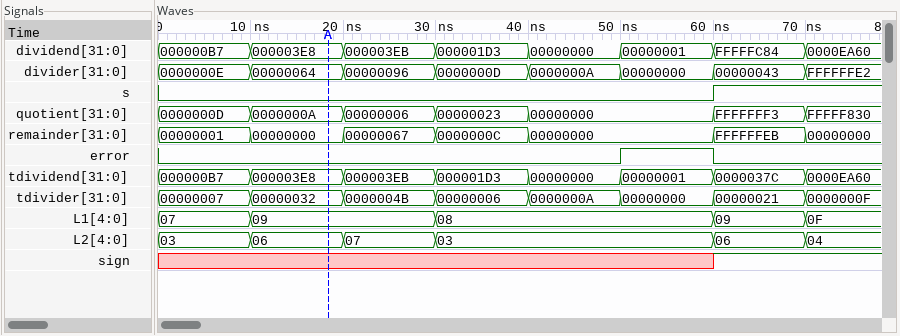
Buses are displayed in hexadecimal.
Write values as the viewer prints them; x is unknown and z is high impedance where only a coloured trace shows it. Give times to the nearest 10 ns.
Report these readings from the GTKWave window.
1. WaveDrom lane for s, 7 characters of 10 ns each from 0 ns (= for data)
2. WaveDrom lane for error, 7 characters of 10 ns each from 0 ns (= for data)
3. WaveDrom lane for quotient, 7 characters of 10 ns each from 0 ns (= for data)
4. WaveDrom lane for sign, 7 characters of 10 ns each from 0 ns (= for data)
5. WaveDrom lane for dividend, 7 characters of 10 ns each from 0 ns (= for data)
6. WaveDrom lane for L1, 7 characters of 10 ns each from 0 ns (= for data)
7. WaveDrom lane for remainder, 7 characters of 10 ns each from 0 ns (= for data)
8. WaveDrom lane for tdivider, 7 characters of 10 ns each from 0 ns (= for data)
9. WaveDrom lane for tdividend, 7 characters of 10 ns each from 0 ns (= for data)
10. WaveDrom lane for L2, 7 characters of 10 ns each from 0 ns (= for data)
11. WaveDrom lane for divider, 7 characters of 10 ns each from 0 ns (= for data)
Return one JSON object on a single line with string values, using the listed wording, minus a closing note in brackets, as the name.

{"WaveDrom lane for s, 7 characters of 10 ns each from 0 ns": "{name: 's', wave: '0.....1'}", "WaveDrom lane for error, 7 characters of 10 ns each from 0 ns": "{name: 'error', wave: '0....10'}", "WaveDrom lane for quotient, 7 characters of 10 ns each from 0 ns": "{name: 'quotient', wave: '=====.=', data: '0000000D 0000000A 00000006 00000023 00000000 FFFFFFF3'}", "WaveDrom lane for sign, 7 characters of 10 ns each from 0 ns": "{name: 'sign', wave: 'x.....1'}", "WaveDrom lane for dividend, 7 characters of 10 ns each from 0 ns": "{name: 'dividend', wave: '=======', data: '000000B7 000003E8 000003EB 000001D3 00000000 00000001 FFFFFC84'}", "WaveDrom lane for L1, 7 characters of 10 ns each from 0 ns": "{name: 'L1', wave: '==.=..=', data: '07 09 08 09'}", "WaveDrom lane for remainder, 7 characters of 10 ns each from 0 ns": "{name: 'remainder', wave: '=====.=', data: '00000001 00000000 00000067 0000000C 00000000 FFFFFFEB'}", "WaveDrom lane for tdivider, 7 characters of 10 ns each from 0 ns": "{name: 'tdivider', wave: '=======', data: '00000007 00000032 0000004B 00000006 0000000A 00000000 00000021'}", "WaveDrom lane for tdividend, 7 characters of 10 ns each from 0 ns": "{name: 'tdividend', wave: '=======', data: '000000B7 000003E8 000003EB 000001D3 00000000 00000001 0000037C'}", "WaveDrom lane for L2, 7 characters of 10 ns each from 0 ns": "{name: 'L2', wave: '====..=', data: '03 06 07 03 06'}", "WaveDrom lane for divider, 7 characters of 10 ns each from 0 ns": "{name: 'divider', wave: '=======', data: '0000000E 00000064 00000096 0000000D 0000000A 00000000 00000043'}"}
